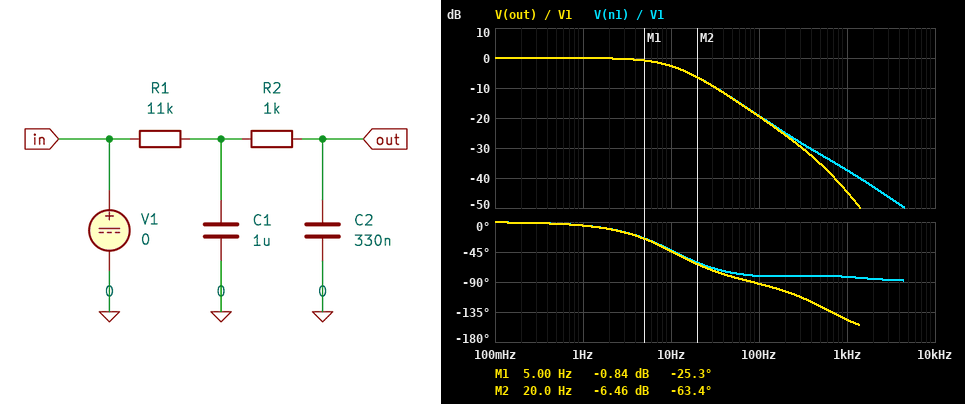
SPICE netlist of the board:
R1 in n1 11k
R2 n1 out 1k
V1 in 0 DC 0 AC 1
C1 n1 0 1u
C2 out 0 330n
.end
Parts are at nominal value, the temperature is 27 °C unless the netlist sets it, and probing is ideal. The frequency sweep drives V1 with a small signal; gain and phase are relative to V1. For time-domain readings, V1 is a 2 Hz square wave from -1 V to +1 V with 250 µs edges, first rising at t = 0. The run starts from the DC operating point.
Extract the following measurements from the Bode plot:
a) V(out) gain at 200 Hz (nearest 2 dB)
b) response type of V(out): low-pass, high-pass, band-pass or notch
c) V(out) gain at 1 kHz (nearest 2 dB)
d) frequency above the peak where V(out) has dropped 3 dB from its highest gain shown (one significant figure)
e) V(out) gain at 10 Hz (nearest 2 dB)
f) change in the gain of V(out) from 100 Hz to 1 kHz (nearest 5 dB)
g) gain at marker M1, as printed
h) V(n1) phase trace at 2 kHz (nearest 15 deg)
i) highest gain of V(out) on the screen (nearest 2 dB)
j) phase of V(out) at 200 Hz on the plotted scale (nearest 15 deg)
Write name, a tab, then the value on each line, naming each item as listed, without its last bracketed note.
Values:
V(out) gain at 200 Hz	-26 dB
response type of V(out): low-pass, high-pass, band-pass or notch	low-pass
V(out) gain at 1 kHz	-44 dB
frequency above the peak where V(out) has dropped 3 dB from its highest gain shown	10 Hz
V(out) gain at 10 Hz	-2 dB
change in the gain of V(out) from 100 Hz to 1 kHz	-25 dB
gain at marker M1, as printed	-0.84 dB
V(n1) phase trace at 2 kHz	-90 deg
highest gain of V(out) on the screen	0 dB
phase of V(out) at 200 Hz on the plotted scale	-105 deg
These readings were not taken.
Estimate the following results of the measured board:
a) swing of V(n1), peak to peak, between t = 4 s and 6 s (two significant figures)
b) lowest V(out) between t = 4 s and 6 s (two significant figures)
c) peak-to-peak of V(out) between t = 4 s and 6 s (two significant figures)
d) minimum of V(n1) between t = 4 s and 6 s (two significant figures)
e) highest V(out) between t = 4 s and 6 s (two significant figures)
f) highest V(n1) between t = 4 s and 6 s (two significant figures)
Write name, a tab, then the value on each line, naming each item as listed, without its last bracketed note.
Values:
swing of V(n1), peak to peak, between t = 4 s and 6 s	2.0 V
lowest V(out) between t = 4 s and 6 s	-1.0 V
peak-to-peak of V(out) between t = 4 s and 6 s	2.0 V
minimum of V(n1) between t = 4 s and 6 s	-1.0 V
highest V(out) between t = 4 s and 6 s	1.0 V
highest V(n1) between t = 4 s and 6 s	1.0 V
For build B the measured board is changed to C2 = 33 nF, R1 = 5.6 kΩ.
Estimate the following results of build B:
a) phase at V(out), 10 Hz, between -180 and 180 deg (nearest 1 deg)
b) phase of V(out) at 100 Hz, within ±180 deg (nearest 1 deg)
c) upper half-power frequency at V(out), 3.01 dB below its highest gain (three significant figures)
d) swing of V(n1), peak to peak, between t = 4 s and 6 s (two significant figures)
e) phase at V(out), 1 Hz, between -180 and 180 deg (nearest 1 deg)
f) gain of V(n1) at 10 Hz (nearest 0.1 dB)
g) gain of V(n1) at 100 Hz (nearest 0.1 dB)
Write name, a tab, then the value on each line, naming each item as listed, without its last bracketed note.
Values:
phase at V(out), 10 Hz, between -180 and 180 deg	-20 deg
phase of V(out) at 100 Hz, within ±180 deg	-76 deg
upper half-power frequency at V(out), 3.01 dB below its highest gain	27.5 Hz
swing of V(n1), peak to peak, between t = 4 s and 6 s	2.0 V
phase at V(out), 1 Hz, between -180 and 180 deg	-2 deg
gain of V(n1) at 10 Hz	-0.5 dB
gain of V(n1) at 100 Hz	-11.5 dB
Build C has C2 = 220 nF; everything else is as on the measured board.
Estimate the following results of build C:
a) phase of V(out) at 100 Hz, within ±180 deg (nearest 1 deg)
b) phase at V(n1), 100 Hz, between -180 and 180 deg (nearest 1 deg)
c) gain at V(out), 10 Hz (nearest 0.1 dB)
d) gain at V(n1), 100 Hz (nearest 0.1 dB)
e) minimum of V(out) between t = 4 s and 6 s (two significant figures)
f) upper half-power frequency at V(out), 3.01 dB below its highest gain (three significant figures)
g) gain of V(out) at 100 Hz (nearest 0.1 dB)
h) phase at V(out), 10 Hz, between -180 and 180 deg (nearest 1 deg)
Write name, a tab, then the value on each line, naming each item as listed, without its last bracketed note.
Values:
phase of V(out) at 100 Hz, within ±180 deg	-90 deg
phase at V(n1), 100 Hz, between -180 and 180 deg	-82 deg
gain at V(out), 10 Hz	-2.3 dB
gain at V(n1), 100 Hz	-18.6 dB
minimum of V(out) between t = 4 s and 6 s	-1.0 V
upper half-power frequency at V(out), 3.01 dB below its highest gain	11.8 Hz
gain of V(out) at 100 Hz	-18.7 dB
phase at V(out), 10 Hz, between -180 and 180 deg	-41 deg
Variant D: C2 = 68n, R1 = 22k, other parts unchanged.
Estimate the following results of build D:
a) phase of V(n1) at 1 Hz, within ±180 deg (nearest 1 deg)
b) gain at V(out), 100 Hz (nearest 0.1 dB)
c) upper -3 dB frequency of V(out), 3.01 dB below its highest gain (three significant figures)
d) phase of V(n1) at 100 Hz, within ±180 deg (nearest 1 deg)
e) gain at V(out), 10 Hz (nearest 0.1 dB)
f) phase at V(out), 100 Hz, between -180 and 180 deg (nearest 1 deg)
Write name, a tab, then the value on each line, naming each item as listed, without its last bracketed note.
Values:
phase of V(n1) at 1 Hz, within ±180 deg	-8 deg
gain at V(out), 100 Hz	-23.4 dB
upper -3 dB frequency of V(out), 3.01 dB below its highest gain	6.77 Hz
phase of V(n1) at 100 Hz, within ±180 deg	-86 deg
gain at V(out), 10 Hz	-5.0 dB
phase at V(out), 100 Hz, between -180 and 180 deg	-88 deg
